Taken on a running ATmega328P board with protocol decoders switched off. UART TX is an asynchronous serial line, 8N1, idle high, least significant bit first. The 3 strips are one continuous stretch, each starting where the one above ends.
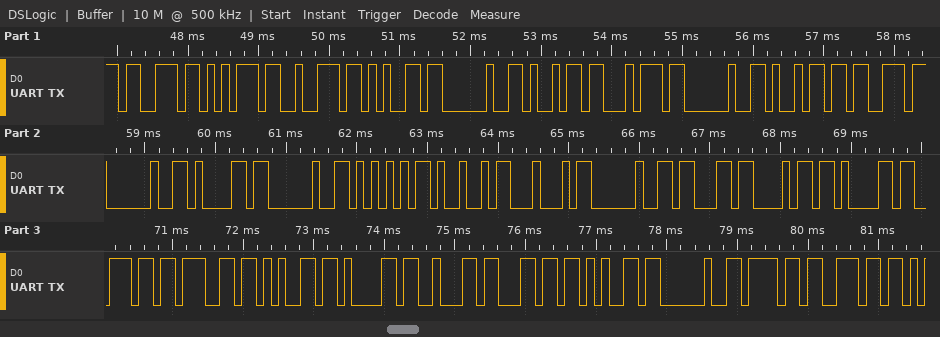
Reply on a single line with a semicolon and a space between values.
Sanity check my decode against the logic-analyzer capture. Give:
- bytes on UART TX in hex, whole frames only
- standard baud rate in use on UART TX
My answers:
0x73 0x75 0x72 0x65 0x20 0x69 0x74 0x20 0x69 0x73 0x20 0x61 0x20 0x55 0x49 0x44 0x20 0x63 0x68 0x61 0x6E 0x67 0x65 0x61 0x62 0x6C 0x65 0x20 0x6F 0x6E; 9600 baud
